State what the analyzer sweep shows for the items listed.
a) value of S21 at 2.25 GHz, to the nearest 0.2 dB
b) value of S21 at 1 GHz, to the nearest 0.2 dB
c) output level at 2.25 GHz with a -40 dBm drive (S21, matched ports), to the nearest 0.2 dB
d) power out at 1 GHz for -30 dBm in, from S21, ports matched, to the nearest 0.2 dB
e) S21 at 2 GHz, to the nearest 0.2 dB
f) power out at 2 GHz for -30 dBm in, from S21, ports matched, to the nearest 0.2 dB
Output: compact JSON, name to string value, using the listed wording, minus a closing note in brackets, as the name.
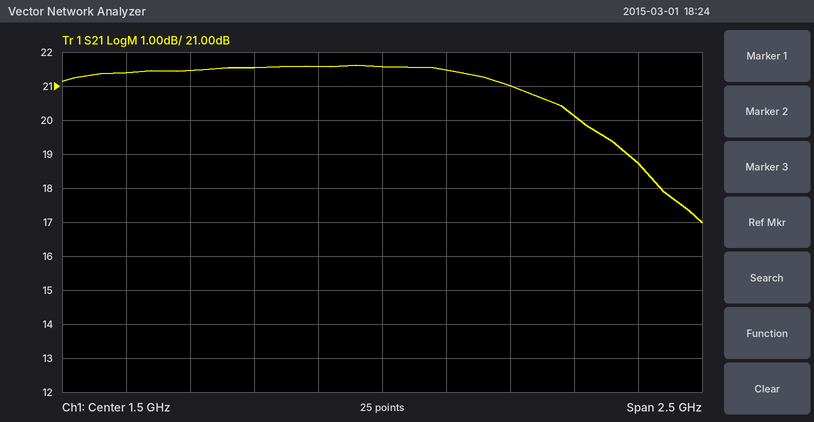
{"value of S21 at 2.25 GHz, to the nearest 0.2 dB": "20.2 dB", "value of S21 at 1 GHz, to the nearest 0.2 dB": "21.6 dB", "output level at 2.25 GHz with a -40 dBm drive (S21, matched ports), to the nearest 0.2 dB": "-19.8 dBm", "power out at 1 GHz for -30 dBm in, from S21, ports matched, to the nearest 0.2 dB": "-8.4 dBm", "S21 at 2 GHz, to the nearest 0.2 dB": "21.0 dB", "power out at 2 GHz for -30 dBm in, from S21, ports matched, to the nearest 0.2 dB": "-9.0 dBm"}
